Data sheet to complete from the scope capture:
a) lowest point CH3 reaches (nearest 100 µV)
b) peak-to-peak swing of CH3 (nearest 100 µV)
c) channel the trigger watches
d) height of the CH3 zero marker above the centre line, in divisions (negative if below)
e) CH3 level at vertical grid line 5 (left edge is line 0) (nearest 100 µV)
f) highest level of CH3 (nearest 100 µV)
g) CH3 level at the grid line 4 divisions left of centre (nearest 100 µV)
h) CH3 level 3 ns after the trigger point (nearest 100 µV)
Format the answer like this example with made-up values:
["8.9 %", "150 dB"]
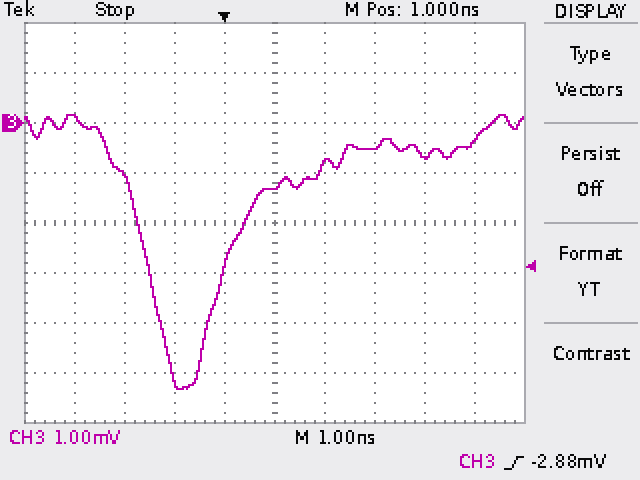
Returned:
["-5.3 mV", "5.5 mV", "CH3", "+2.0 div", "-1.3 mV", "200 µV", "100 µV", "-500 µV"]
